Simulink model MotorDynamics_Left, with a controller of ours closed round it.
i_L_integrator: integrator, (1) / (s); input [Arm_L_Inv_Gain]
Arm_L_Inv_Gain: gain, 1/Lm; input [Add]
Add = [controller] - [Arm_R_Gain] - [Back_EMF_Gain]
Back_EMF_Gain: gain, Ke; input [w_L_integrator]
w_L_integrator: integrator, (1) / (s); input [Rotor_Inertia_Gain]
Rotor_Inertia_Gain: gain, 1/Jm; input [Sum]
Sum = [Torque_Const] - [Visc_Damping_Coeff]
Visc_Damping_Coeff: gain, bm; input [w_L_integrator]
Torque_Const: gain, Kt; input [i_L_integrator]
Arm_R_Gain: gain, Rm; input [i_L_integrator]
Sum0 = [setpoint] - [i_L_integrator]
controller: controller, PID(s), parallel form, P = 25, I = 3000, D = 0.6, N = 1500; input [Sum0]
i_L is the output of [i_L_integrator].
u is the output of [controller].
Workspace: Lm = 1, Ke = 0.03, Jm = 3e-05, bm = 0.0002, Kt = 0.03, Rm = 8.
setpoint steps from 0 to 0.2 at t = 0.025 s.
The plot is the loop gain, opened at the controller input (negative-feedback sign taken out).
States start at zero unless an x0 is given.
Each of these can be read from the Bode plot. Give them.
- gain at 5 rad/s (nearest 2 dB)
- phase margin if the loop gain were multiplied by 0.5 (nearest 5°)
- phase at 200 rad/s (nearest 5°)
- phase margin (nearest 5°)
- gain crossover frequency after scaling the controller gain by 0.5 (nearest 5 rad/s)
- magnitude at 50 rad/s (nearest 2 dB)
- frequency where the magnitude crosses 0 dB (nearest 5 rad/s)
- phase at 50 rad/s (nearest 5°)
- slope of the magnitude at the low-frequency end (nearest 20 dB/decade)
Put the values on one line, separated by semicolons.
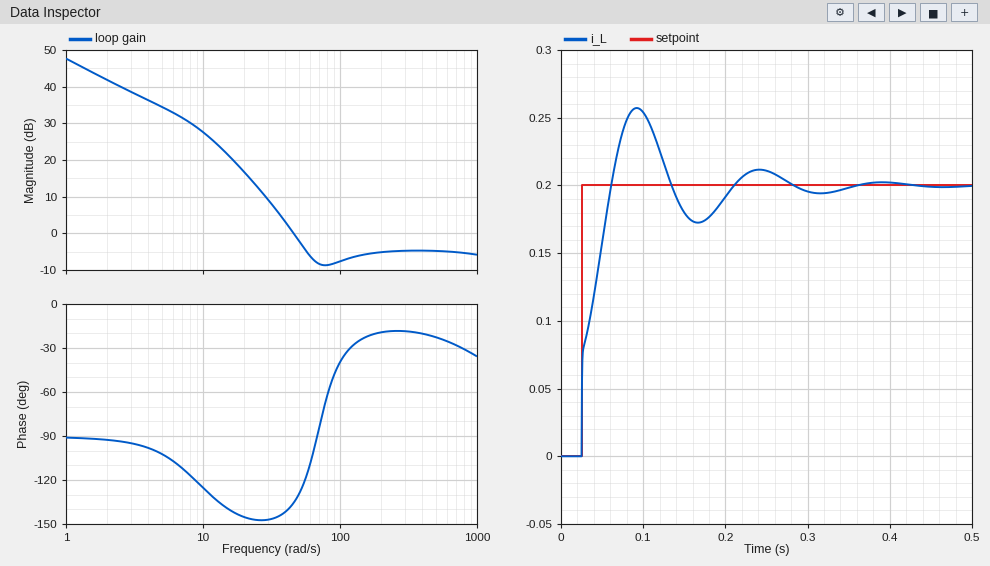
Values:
34 dB; 35°; -20°; 45°; 35 rad/s; -2 dB; 45 rad/s; -130°; -20 dB/decade
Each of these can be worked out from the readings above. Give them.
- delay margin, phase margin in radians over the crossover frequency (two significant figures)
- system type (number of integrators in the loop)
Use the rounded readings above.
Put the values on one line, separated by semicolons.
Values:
0.017 s; 1
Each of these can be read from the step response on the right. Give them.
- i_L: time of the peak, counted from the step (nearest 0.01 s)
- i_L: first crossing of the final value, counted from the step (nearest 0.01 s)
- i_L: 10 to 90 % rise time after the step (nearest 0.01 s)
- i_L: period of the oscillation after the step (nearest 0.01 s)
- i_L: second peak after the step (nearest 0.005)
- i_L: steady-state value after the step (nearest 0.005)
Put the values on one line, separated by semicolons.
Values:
0.07 s; 0.04 s; 0.03 s; 0.15 s; 0.210; 0.200
